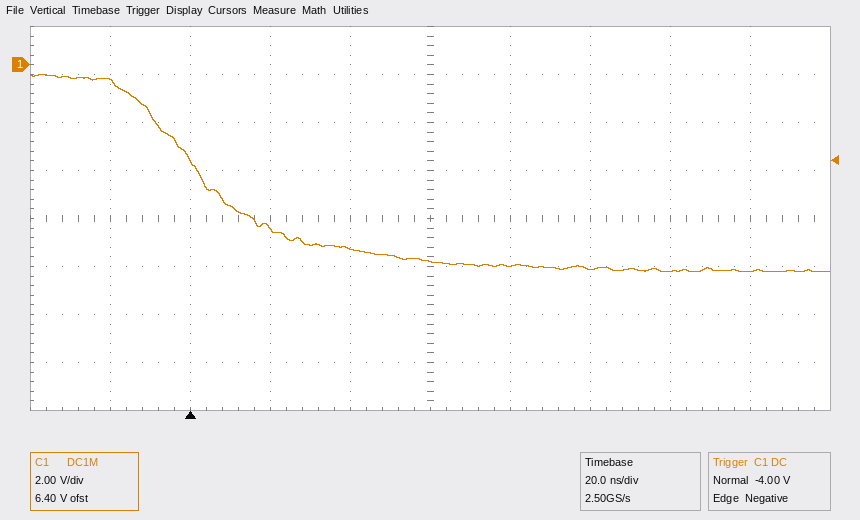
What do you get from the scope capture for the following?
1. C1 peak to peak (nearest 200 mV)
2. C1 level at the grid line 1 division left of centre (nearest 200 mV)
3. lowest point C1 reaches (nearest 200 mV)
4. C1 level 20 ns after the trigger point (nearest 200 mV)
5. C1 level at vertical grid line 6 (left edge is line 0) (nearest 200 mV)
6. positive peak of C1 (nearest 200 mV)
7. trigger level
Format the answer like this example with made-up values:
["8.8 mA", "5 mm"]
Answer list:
["8.2 V", "-7.6 V", "-8.6 V", "-6.8 V", "-8.4 V", "-400 mV", "-4.00 V"]
